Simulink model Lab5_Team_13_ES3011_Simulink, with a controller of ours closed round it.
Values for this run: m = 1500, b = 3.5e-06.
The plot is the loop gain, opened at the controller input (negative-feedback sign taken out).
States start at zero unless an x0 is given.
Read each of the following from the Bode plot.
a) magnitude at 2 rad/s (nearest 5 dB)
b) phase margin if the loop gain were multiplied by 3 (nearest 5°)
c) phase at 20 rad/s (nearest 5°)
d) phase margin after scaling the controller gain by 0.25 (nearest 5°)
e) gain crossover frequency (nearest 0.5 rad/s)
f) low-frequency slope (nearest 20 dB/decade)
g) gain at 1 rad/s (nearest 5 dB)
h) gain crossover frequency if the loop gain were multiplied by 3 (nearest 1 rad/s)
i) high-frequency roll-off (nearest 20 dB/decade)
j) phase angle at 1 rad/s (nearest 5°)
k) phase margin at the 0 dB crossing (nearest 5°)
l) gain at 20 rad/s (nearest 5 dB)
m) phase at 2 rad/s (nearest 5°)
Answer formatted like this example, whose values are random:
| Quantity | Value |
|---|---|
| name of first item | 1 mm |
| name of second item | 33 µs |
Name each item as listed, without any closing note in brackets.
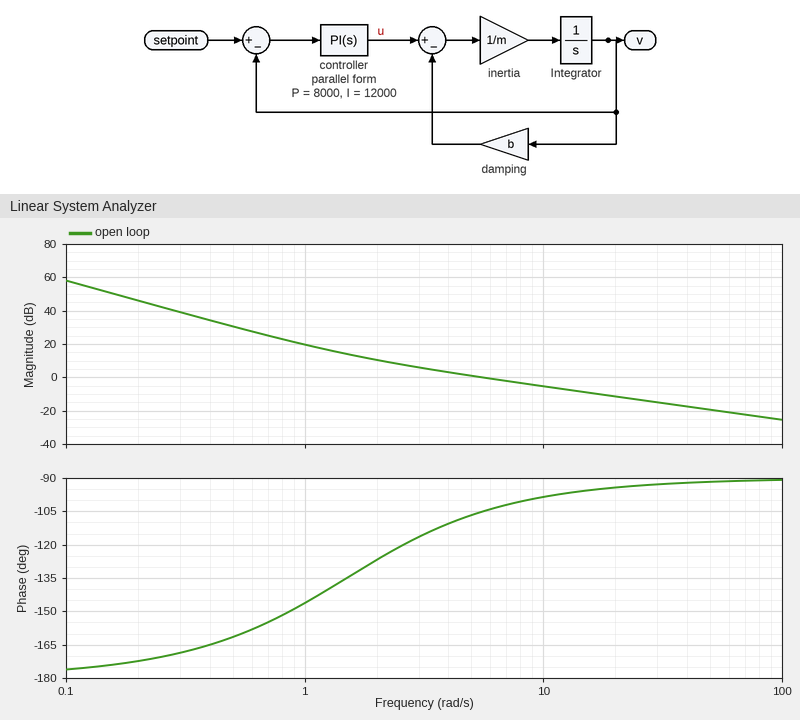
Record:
| Quantity | Value |
|---|---|
| magnitude at 2 rad/s | 10 dB |
| phase margin if the loop gain were multiplied by 3 | 85° |
| phase at 20 rad/s | -95° |
| phase margin after scaling the controller gain by 0.25 | 50° |
| gain crossover frequency | 5.5 rad/s |
| low-frequency slope | -40 dB/decade |
| gain at 1 rad/s | 20 dB |
| gain crossover frequency if the loop gain were multiplied by 3 | 16 rad/s |
| high-frequency roll-off | -20 dB/decade |
| phase angle at 1 rad/s | -145° |
| phase margin at the 0 dB crossing | 75° |
| gain at 20 rad/s | -10 dB |
| phase at 2 rad/s | -125° |
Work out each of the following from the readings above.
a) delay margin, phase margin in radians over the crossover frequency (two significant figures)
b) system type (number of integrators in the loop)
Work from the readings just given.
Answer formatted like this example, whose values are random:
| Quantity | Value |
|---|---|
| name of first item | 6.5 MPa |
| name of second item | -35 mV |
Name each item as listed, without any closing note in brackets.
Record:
| Quantity | Value |
|---|---|
| delay margin, phase margin in radians over the crossover frequency | 0.24 s |
| system type | 2 |
